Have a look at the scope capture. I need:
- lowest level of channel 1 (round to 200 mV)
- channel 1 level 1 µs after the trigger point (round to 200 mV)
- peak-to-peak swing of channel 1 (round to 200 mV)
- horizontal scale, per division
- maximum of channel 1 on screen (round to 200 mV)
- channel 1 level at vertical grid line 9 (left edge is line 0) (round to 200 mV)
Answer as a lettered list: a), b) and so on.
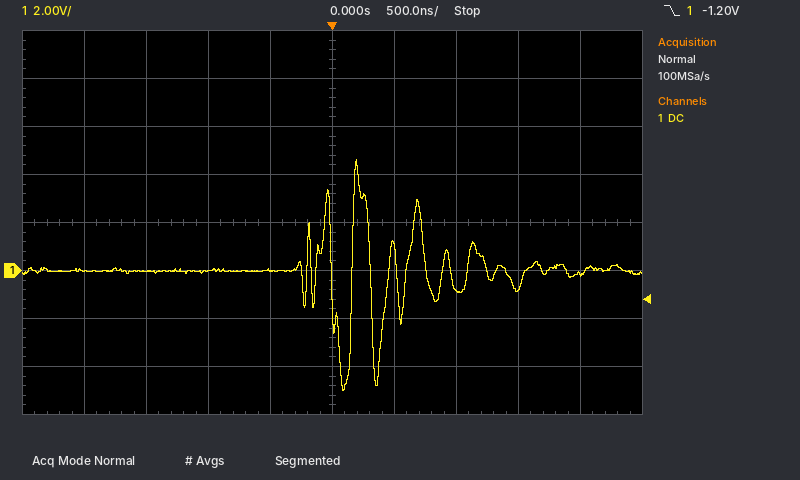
a) -5.0 V
b) -800 mV
c) 9.6 V
d) 500 ns
e) 4.6 V
f) -200 mV
